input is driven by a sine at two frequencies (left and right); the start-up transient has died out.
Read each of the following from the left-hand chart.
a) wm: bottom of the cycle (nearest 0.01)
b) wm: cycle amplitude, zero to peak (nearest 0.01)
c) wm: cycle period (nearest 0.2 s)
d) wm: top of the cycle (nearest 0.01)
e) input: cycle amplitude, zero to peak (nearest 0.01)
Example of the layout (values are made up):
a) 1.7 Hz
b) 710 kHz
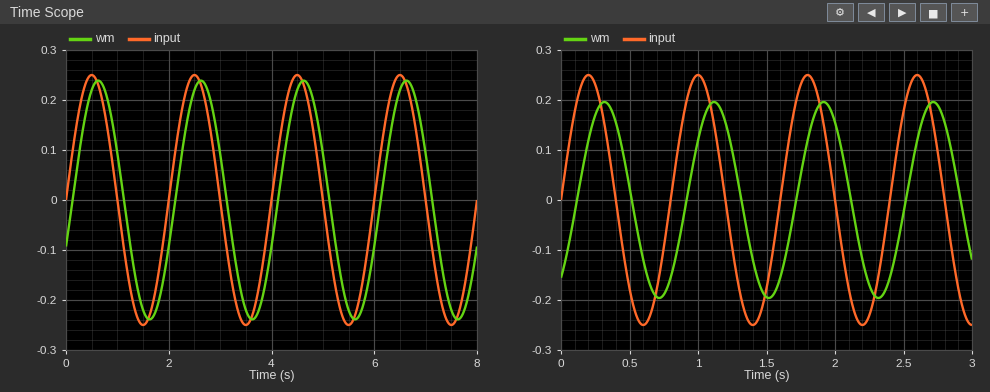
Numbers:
a) -0.24
b) 0.24
c) 2.0 s
d) 0.24
e) 0.25
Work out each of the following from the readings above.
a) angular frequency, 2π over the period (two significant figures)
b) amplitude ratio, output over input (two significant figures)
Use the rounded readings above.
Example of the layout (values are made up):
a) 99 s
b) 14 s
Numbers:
a) 3.1 rad/s
b) 0.96
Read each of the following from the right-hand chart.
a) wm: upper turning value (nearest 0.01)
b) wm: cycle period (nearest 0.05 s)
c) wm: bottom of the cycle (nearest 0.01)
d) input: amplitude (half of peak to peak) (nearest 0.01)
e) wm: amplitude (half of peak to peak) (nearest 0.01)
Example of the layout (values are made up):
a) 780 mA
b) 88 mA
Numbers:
a) 0.20
b) 0.80 s
c) -0.20
d) 0.25
e) 0.20
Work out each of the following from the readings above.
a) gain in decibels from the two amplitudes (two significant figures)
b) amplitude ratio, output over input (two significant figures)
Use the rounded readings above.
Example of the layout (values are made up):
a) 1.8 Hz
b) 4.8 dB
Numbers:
a) -1.9 dB
b) 0.80
